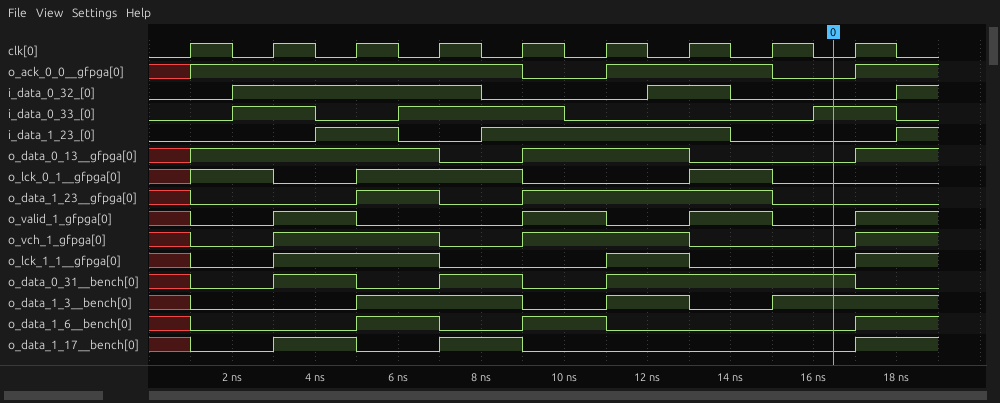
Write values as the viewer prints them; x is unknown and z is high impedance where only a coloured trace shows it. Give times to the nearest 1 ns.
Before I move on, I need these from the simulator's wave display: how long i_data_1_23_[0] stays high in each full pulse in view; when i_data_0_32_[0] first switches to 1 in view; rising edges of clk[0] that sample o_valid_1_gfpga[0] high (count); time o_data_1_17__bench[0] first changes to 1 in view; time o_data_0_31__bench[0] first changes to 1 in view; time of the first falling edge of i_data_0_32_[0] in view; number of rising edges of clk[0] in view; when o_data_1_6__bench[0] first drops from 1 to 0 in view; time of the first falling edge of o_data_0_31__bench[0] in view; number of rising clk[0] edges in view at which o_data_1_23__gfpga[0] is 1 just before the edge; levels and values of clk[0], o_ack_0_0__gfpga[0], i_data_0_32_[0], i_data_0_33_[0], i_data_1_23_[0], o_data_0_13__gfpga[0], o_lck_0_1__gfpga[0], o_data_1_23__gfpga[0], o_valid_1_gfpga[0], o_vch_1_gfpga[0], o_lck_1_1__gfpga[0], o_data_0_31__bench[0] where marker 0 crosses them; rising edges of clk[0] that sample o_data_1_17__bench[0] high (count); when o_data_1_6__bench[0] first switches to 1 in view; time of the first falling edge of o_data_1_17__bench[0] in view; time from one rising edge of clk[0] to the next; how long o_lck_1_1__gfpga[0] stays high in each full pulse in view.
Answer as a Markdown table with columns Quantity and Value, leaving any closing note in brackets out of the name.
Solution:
| Quantity | Value |
|---|---|
| how long i_data_1_23_[0] stays high in each full pulse in view | 2 ns, 6 ns |
| when i_data_0_32_[0] first switches to 1 in view | 2 ns |
| rising edges of clk[0] that sample o_valid_1_gfpga[0] high | 3 |
| time o_data_1_17__bench[0] first changes to 1 in view | 3 ns |
| time o_data_0_31__bench[0] first changes to 1 in view | 3 ns |
| time of the first falling edge of i_data_0_32_[0] in view | 8 ns |
| number of rising edges of clk[0] in view | 9 |
| when o_data_1_6__bench[0] first drops from 1 to 0 in view | 7 ns |
| time of the first falling edge of o_data_0_31__bench[0] in view | 5 ns |
| number of rising clk[0] edges in view at which o_data_1_23__gfpga[0] is 1 just before the edge | 4 |
| levels and values of clk[0], o_ack_0_0__gfpga[0], i_data_0_32_[0], i_data_0_33_[0], i_data_1_23_[0], o_data_0_13__gfpga[0], o_lck_0_1__gfpga[0], o_data_1_23__gfpga[0], o_valid_1_gfpga[0], o_vch_1_gfpga[0], o_lck_1_1__gfpga[0], o_data_0_31__bench[0] where marker 0 crosses them | clk[0]=0, o_ack_0_0__gfpga[0]=0, i_data_0_32_[0]=0, i_data_0_33_[0]=1, i_data_1_23_[0]=0, o_data_0_13__gfpga[0]=0, o_lck_0_1__gfpga[0]=0, o_data_1_23__gfpga[0]=0, o_valid_1_gfpga[0]=0, o_vch_1_gfpga[0]=0, o_lck_1_1__gfpga[0]=0, o_data_0_31__bench[0]=1 |
| rising edges of clk[0] that sample o_data_1_17__bench[0] high | 2 |
| when o_data_1_6__bench[0] first switches to 1 in view | 5 ns |
| time of the first falling edge of o_data_1_17__bench[0] in view | 5 ns |
| time from one rising edge of clk[0] to the next | 2 ns |
| how long o_lck_1_1__gfpga[0] stays high in each full pulse in view | 4 ns, 2 ns |
